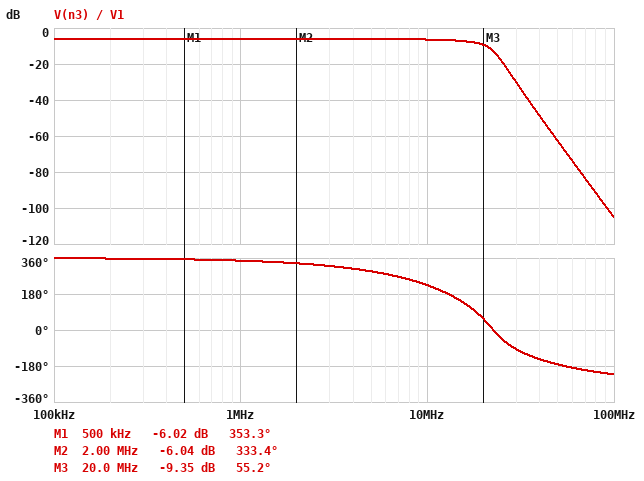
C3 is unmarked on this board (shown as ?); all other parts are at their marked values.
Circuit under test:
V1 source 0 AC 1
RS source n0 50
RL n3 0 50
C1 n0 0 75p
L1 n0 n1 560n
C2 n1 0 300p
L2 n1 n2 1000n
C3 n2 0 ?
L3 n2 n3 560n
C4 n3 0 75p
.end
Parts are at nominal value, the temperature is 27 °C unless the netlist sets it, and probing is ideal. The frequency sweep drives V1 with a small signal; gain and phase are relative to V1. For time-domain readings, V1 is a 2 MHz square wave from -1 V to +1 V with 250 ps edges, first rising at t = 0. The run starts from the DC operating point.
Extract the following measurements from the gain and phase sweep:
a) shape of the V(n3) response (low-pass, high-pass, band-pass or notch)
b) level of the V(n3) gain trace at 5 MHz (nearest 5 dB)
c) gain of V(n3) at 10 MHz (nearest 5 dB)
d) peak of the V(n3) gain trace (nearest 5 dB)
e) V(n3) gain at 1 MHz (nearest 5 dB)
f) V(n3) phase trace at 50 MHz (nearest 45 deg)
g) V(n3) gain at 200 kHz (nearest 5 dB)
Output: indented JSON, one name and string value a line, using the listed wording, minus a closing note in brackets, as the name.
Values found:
{
  "shape of the V(n3) response": "low-pass",
  "level of the V(n3) gain trace at 5 MHz": "-5 dB",
  "gain of V(n3) at 10 MHz": "-5 dB",
  "peak of the V(n3) gain trace": "-5 dB",
  "V(n3) gain at 1 MHz": "-5 dB",
  "V(n3) phase trace at 50 MHz": "-180 deg",
  "V(n3) gain at 200 kHz": "-5 dB"
}
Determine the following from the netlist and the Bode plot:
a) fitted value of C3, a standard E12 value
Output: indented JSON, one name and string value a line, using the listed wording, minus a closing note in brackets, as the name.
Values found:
{
  "fitted value of C3, a standard E12 value": "180 pF"
}
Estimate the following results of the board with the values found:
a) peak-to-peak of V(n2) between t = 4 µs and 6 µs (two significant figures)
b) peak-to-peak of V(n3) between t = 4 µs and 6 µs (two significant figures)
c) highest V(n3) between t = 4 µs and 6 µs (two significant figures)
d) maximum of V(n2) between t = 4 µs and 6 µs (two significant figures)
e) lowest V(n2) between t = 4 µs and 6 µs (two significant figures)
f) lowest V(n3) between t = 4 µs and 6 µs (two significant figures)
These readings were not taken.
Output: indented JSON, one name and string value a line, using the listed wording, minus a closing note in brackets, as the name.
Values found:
{
  "peak-to-peak of V(n2) between t = 4 µs and 6 µs": "1.4 V",
  "peak-to-peak of V(n3) between t = 4 µs and 6 µs": "1.2 V",
  "highest V(n3) between t = 4 µs and 6 µs": "620 mV",
  "maximum of V(n2) between t = 4 µs and 6 µs": "690 mV",
  "lowest V(n2) between t = 4 µs and 6 µs": "-690 mV",
  "lowest V(n3) between t = 4 µs and 6 µs": "-620 mV"
}
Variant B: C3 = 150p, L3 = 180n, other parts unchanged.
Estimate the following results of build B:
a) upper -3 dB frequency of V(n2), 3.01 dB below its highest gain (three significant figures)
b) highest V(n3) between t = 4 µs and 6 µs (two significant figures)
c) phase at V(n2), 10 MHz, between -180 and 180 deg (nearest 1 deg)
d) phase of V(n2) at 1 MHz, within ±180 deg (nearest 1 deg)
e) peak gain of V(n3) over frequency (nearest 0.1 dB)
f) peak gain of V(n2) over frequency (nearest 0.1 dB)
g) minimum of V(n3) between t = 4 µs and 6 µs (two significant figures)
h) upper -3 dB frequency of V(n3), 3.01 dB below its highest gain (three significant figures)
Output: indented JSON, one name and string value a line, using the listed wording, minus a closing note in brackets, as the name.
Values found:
{
  "upper -3 dB frequency of V(n2), 3.01 dB below its highest gain": "16.3 MHz",
  "highest V(n3) between t = 4 µs and 6 µs": "610 mV",
  "phase at V(n2), 10 MHz, between -180 and 180 deg": "-108 deg",
  "phase of V(n2) at 1 MHz, within ±180 deg": "-10 deg",
  "peak gain of V(n3) over frequency": "-6.0 dB",
  "peak gain of V(n2) over frequency": "-6.0 dB",
  "minimum of V(n3) between t = 4 µs and 6 µs": "-610 mV",
  "upper -3 dB frequency of V(n3), 3.01 dB below its highest gain": "17.0 MHz"
}
